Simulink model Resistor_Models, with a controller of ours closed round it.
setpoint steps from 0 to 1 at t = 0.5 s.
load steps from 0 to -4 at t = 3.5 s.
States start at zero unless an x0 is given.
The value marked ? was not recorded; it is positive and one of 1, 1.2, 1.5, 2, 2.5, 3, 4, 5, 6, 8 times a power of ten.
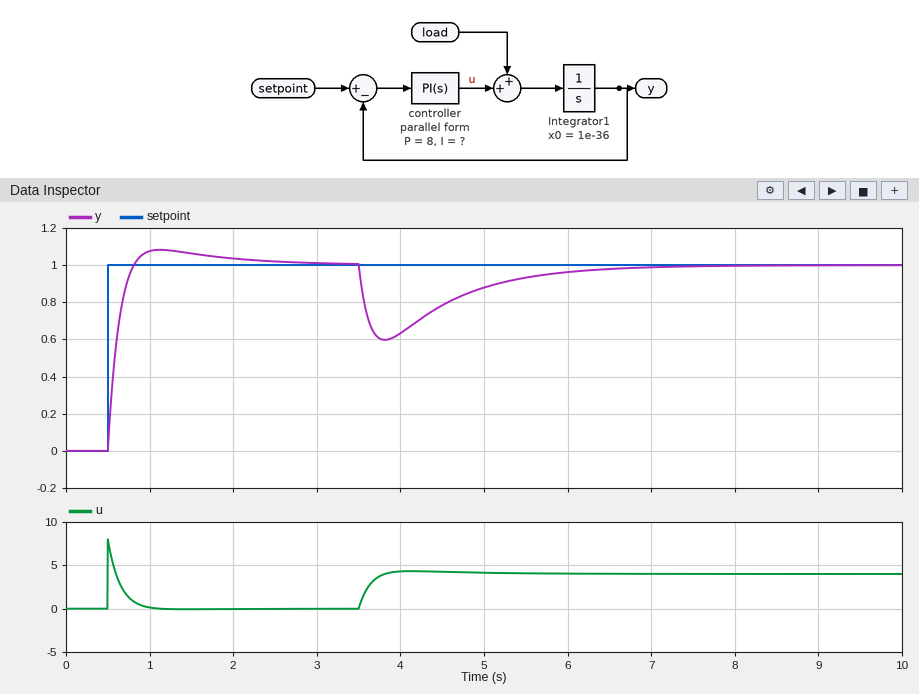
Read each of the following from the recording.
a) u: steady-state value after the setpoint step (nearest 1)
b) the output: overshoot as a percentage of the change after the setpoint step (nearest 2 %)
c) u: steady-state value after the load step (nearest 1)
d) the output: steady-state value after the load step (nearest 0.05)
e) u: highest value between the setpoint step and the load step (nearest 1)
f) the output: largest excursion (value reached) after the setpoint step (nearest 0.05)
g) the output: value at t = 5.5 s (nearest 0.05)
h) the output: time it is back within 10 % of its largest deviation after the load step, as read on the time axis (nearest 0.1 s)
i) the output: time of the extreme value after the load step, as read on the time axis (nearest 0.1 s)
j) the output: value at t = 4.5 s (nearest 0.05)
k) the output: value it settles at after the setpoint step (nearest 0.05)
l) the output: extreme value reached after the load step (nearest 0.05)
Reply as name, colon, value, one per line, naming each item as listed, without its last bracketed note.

u: steady-state value after the setpoint step: 0
the output: overshoot as a percentage of the change after the setpoint step: 8 %
u: steady-state value after the load step: 4
the output: steady-state value after the load step: 1.00
u: highest value between the setpoint step and the load step: 8
the output: largest excursion (value reached) after the setpoint step: 1.10
the output: value at t = 5.5 s: 0.95
the output: time it is back within 10 % of its largest deviation after the load step, as read on the time axis: 5.9 s
the output: time of the extreme value after the load step, as read on the time axis: 3.8 s
the output: value at t = 4.5 s: 0.80
the output: value it settles at after the setpoint step: 1.00
the output: extreme value reached after the load step: 0.60
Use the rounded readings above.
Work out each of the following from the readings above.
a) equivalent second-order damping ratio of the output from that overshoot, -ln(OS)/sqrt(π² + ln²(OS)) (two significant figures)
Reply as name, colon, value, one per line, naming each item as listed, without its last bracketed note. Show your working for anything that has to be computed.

equivalent second-order damping ratio of the output from that overshoot, -ln(OS)/sqrt(π² + ln²(OS)): ln(0.08) = -2.526; 2.526 / sqrt(9.870 + 6.379) = 0.63
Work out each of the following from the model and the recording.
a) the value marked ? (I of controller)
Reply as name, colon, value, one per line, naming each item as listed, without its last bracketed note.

the value marked ?: 8
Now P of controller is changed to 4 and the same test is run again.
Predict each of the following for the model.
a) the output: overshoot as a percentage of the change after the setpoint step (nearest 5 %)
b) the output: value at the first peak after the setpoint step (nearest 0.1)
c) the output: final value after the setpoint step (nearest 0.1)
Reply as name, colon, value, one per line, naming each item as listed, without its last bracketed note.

the output: overshoot as a percentage of the change after the setpoint step: 20 %
the output: value at the first peak after the setpoint step: 1.2
the output: final value after the setpoint step: 1.0
